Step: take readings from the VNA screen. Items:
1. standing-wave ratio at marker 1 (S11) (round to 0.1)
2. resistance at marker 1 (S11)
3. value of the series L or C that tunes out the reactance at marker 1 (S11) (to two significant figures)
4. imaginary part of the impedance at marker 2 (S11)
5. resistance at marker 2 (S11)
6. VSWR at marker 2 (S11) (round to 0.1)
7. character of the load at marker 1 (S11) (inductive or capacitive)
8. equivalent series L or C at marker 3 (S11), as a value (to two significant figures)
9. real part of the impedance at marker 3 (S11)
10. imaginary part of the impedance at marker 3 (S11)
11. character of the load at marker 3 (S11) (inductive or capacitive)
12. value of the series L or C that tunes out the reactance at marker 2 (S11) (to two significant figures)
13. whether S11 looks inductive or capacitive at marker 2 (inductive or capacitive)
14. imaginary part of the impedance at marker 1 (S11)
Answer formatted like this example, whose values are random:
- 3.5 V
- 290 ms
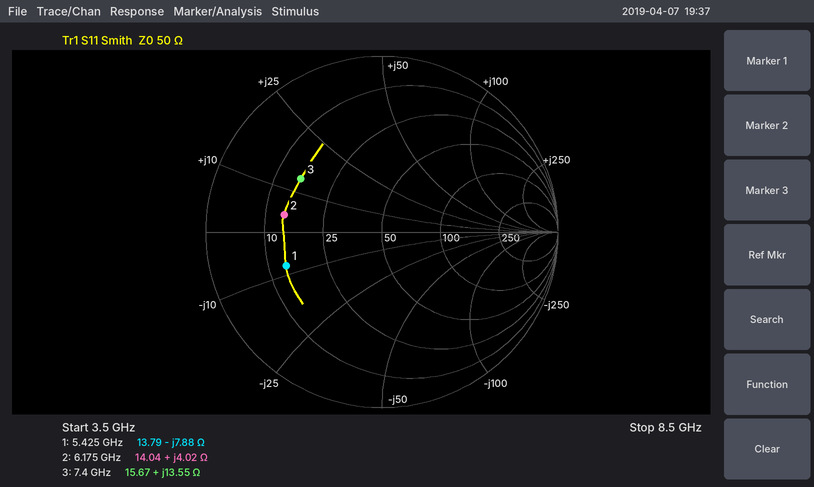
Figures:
- 3.7
- 13.79 Ω
- 230 pH
- +4.02 Ω
- 14.04 Ω
- 3.6
- capacitive
- 290 pH
- 15.67 Ω
- +13.55 Ω
- inductive
- 6.4 pF
- inductive
- -7.88 Ω
